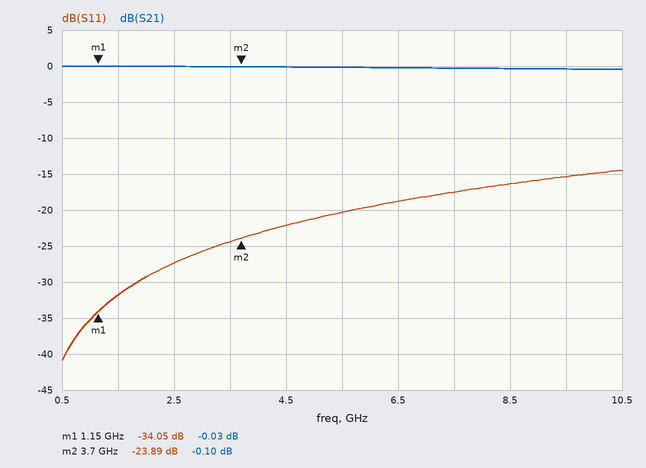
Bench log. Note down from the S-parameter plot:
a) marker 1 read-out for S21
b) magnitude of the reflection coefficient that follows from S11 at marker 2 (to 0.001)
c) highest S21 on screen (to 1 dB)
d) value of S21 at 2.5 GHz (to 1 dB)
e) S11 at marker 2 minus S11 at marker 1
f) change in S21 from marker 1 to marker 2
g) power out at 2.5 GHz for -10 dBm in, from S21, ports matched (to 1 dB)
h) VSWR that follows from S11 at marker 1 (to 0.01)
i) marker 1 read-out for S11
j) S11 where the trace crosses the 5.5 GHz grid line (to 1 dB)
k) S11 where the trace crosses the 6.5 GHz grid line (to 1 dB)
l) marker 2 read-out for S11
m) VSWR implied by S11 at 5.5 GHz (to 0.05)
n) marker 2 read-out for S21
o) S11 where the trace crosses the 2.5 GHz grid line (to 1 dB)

-0.03 dB
0.064
0 dB
0 dB
10.16 dB
-0.07 dB
-10 dBm
1.04
-34.05 dB
-20 dB
-19 dB
-23.89 dB
1.20
-0.10 dB
-27 dB
